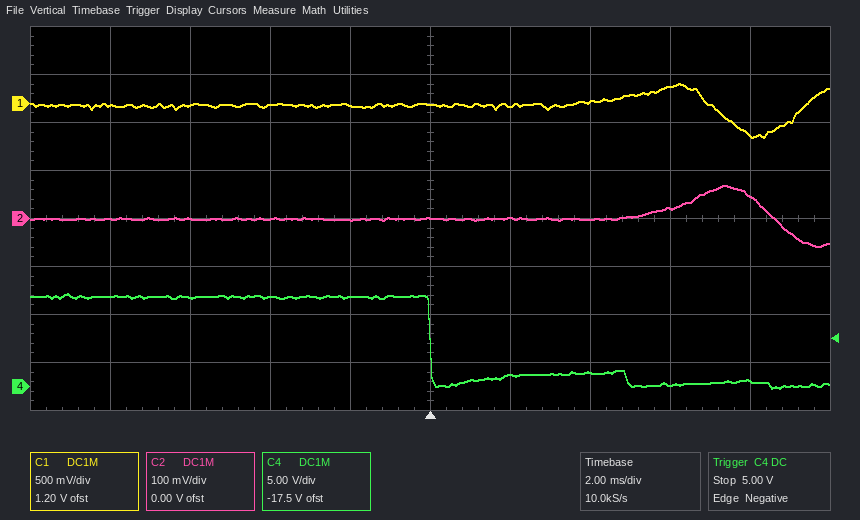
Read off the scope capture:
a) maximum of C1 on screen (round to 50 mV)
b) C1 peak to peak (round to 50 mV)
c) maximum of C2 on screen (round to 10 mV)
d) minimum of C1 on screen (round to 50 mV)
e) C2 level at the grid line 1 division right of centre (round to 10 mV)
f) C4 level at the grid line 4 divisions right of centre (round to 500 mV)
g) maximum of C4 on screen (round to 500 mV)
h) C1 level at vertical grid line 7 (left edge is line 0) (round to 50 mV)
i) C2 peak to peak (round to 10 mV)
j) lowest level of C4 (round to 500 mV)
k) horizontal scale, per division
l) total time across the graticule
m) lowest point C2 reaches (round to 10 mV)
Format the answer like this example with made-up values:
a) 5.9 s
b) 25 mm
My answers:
a) 200 mV
b) 550 mV
c) 70 mV
d) -350 mV
e) 0 mV
f) 500 mV
g) 9.5 V
h) 0 mV
i) 130 mV
j) 0.0 V
k) 2 ms
l) 20 ms
m) -60 mV
